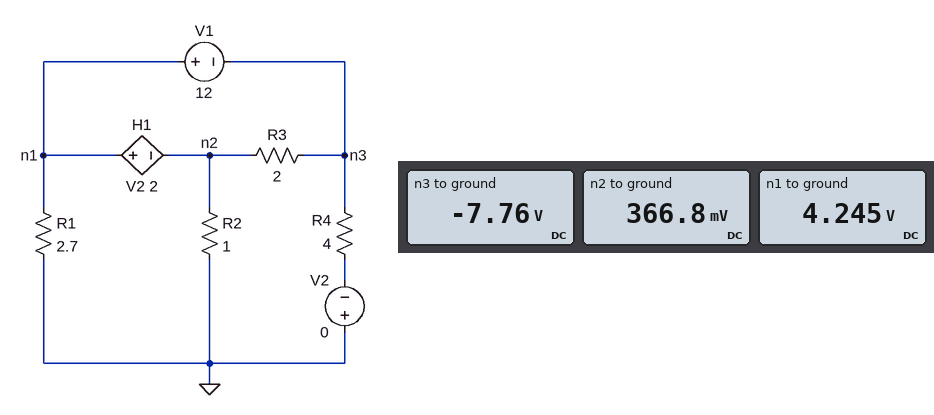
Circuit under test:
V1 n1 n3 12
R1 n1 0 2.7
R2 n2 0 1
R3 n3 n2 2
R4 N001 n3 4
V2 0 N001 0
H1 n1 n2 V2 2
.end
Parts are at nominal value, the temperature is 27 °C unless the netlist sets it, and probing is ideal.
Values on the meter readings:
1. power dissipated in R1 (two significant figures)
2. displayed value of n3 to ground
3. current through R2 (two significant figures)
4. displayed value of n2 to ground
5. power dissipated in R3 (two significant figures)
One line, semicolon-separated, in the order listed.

6.7 W; -7.76 V; 370 mA; 366.8 mV; 33 W
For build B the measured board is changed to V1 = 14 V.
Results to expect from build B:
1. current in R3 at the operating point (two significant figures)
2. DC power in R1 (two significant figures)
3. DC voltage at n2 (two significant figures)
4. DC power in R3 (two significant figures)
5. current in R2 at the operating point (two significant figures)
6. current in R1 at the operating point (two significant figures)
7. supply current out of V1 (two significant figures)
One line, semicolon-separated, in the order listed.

4.7 A; 9.1 W; 430 mV; 45 W; 430 mA; 1.8 A; 7.0 A
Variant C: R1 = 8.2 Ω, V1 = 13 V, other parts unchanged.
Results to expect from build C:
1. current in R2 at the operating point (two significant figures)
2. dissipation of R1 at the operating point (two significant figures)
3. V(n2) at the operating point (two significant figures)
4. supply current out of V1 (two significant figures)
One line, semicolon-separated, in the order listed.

1.3 A; 3.3 W; 1.3 V; 6.5 A
